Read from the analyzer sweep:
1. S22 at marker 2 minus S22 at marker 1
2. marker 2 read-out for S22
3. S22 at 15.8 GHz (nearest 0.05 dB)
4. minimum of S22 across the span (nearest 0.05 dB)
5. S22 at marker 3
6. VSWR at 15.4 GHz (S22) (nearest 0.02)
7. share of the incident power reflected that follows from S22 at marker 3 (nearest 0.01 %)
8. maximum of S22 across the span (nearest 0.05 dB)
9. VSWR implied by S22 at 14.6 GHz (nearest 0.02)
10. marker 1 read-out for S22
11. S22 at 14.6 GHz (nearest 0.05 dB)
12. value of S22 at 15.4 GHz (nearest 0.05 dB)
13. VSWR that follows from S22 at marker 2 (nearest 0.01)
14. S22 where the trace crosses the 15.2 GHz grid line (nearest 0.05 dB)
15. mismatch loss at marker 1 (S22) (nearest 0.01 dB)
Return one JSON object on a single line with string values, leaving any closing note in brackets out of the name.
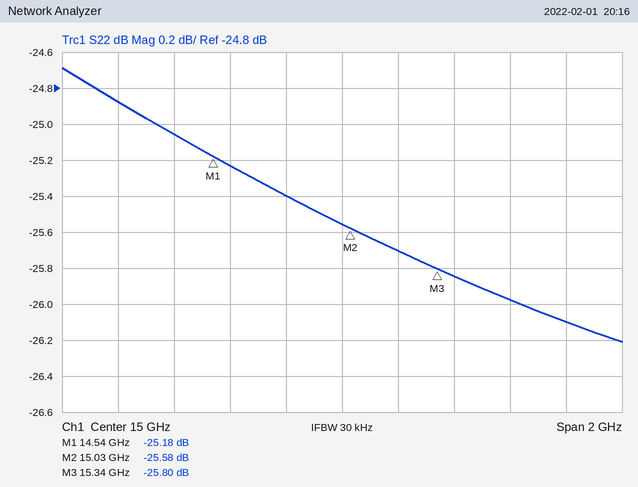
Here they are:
{"S22 at marker 2 minus S22 at marker 1": "-0.40 dB", "marker 2 read-out for S22": "-25.58 dB", "S22 at 15.8 GHz": "-26.10 dB", "minimum of S22 across the span": "-26.20 dB", "S22 at marker 3": "-25.80 dB", "VSWR at 15.4 GHz (S22)": "1.10", "share of the incident power reflected that follows from S22 at marker 3": "0.26 %", "maximum of S22 across the span": "-24.70 dB", "VSWR implied by S22 at 14.6 GHz": "1.12", "marker 1 read-out for S22": "-25.18 dB", "S22 at 14.6 GHz": "-25.25 dB", "value of S22 at 15.4 GHz": "-25.85 dB", "VSWR that follows from S22 at marker 2": "1.11", "S22 where the trace crosses the 15.2 GHz grid line": "-25.70 dB", "mismatch loss at marker 1 (S22)": "0.01 dB"}
